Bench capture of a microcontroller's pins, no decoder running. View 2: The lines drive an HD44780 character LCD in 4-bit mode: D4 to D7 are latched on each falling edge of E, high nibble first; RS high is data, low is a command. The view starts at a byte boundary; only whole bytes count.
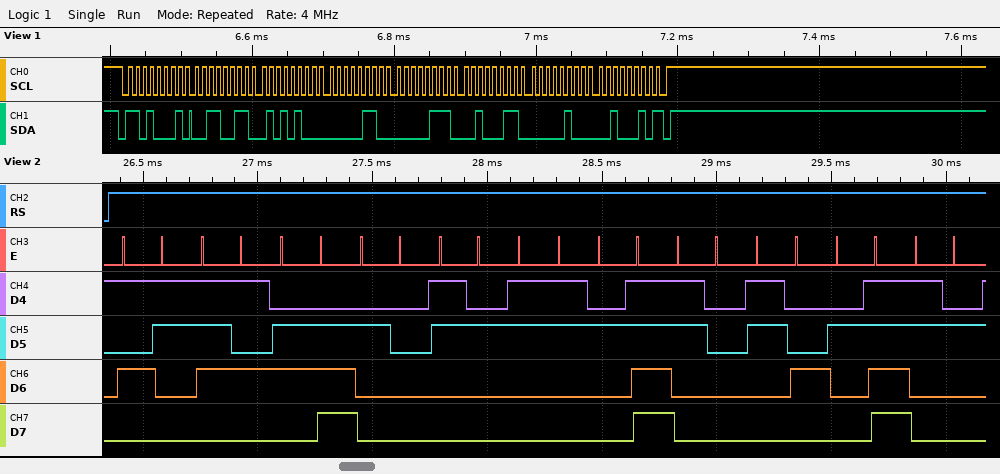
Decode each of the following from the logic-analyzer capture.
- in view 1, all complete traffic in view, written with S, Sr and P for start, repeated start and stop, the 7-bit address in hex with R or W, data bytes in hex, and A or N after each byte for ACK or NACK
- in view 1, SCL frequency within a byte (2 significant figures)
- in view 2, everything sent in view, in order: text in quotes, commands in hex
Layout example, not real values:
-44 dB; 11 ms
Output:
S 68R A 33 A 54 A 06 A 07 A 23 A 04 A 22 N P; 100 kHz; "Sun 23/04/2"
